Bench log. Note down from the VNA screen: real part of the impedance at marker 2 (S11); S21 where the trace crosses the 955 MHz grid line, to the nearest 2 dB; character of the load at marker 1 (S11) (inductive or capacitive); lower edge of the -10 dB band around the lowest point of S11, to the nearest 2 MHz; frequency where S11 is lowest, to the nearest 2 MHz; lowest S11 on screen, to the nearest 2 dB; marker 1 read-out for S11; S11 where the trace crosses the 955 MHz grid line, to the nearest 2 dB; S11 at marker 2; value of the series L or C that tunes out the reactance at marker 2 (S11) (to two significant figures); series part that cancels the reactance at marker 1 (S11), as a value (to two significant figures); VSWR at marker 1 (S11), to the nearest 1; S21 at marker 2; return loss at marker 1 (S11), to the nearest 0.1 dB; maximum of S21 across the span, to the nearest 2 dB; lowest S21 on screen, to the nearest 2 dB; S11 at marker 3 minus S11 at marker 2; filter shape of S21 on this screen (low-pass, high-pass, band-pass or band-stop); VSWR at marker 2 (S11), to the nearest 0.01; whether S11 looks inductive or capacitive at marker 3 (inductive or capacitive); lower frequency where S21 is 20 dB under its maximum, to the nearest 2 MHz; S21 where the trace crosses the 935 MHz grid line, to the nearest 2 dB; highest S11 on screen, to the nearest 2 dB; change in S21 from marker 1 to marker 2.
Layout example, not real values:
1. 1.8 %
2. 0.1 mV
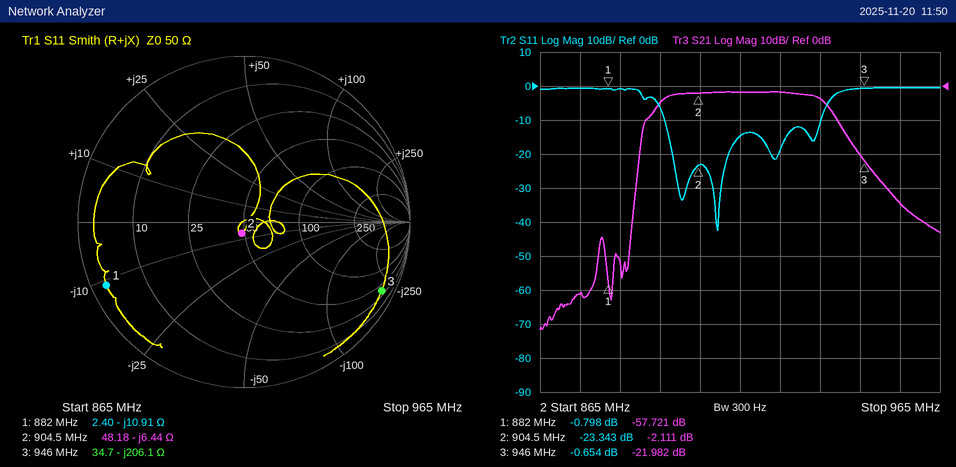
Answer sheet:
1. 48.18 Ω
2. -34 dB
3. capacitive
4. 896 MHz
5. 910 MHz
6. -42 dB
7. -0.798 dB
8. 0 dB
9. -23.343 dB
10. 1.1 nH
11. 2.0 nH
12. 22
13. -2.111 dB
14. 0.8 dB
15. -2 dB
16. -72 dB
17. 22.689 dB
18. band-pass
19. 1.15
20. capacitive
21. 890 MHz
22. -4 dB
23. 0 dB
24. 55.610 dB
